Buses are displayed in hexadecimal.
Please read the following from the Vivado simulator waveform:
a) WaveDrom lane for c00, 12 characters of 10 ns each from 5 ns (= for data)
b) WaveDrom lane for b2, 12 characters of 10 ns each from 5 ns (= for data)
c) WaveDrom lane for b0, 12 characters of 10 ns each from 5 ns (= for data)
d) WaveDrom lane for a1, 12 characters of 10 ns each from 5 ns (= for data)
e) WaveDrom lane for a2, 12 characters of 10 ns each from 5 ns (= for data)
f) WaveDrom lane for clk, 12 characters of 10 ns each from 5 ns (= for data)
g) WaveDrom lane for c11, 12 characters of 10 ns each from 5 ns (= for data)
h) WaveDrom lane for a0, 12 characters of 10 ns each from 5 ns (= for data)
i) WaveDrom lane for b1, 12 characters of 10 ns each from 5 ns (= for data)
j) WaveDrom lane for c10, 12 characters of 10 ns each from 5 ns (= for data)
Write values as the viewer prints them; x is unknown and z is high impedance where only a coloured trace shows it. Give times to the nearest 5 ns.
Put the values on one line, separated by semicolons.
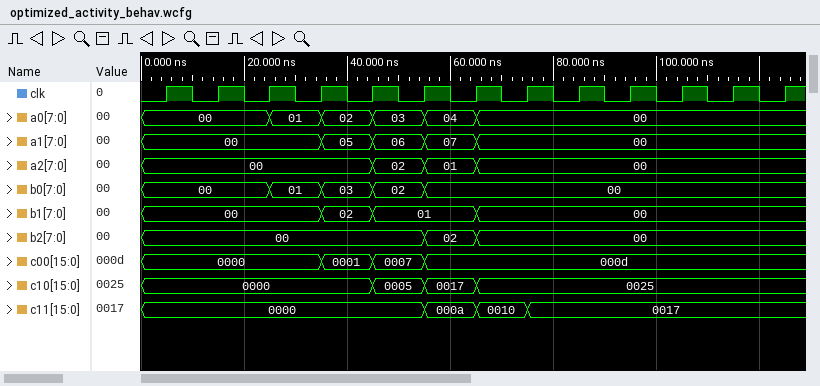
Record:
{name: 'c00', wave: '=..===......', data: '0000 0001 0007 000d'}; {name: 'b2', wave: '=....==.....', data: '00 02 00'}; {name: 'b0', wave: '=.====......', data: '00 01 03 02 00'}; {name: 'a1', wave: '=..====.....', data: '00 05 06 07 00'}; {name: 'a2', wave: '=...===.....', data: '00 02 01 00'}; {name: 'clk', wave: 'p...........'}; {name: 'c11', wave: '=....===....', data: '0000 000a 0010 0017'}; {name: 'a0', wave: '=.=====.....', data: '00 01 02 03 04 00'}; {name: 'b1', wave: '=..==.=.....', data: '00 02 01 00'}; {name: 'c10', wave: '=...===.....', data: '0000 0005 0017 0025'}
